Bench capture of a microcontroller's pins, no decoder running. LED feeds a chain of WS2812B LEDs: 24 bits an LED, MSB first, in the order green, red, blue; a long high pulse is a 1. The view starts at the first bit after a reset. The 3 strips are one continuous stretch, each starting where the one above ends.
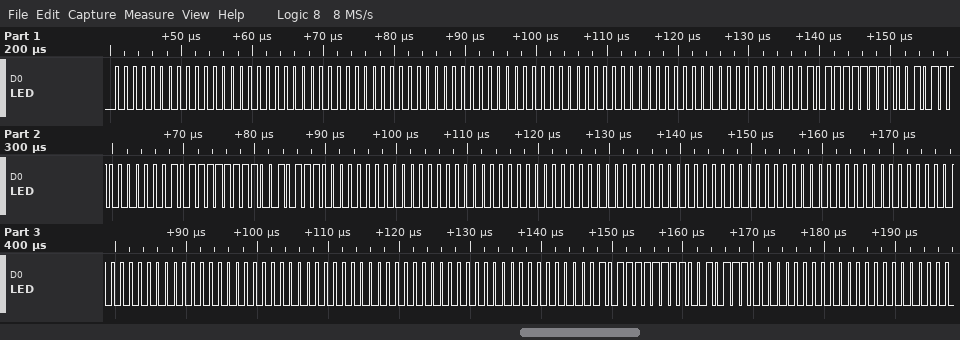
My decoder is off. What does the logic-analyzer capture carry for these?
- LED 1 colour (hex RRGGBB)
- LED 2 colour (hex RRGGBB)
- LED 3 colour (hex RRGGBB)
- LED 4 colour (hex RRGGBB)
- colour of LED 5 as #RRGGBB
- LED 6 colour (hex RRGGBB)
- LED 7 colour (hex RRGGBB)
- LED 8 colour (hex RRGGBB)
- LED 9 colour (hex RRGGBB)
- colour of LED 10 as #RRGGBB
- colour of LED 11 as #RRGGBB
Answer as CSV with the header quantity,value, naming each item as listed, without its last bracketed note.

quantity,value
LED 1 colour,#000000
LED 2 colour,#000000
LED 3 colour,#000000
LED 4 colour,#FF022E
colour of LED 5 as #RRGGBB,#FF022E
LED 6 colour,#000000
LED 7 colour,#000000
LED 8 colour,#000000
LED 9 colour,#000000
colour of LED 10 as #RRGGBB,#000000
colour of LED 11 as #RRGGBB,#FF022E
